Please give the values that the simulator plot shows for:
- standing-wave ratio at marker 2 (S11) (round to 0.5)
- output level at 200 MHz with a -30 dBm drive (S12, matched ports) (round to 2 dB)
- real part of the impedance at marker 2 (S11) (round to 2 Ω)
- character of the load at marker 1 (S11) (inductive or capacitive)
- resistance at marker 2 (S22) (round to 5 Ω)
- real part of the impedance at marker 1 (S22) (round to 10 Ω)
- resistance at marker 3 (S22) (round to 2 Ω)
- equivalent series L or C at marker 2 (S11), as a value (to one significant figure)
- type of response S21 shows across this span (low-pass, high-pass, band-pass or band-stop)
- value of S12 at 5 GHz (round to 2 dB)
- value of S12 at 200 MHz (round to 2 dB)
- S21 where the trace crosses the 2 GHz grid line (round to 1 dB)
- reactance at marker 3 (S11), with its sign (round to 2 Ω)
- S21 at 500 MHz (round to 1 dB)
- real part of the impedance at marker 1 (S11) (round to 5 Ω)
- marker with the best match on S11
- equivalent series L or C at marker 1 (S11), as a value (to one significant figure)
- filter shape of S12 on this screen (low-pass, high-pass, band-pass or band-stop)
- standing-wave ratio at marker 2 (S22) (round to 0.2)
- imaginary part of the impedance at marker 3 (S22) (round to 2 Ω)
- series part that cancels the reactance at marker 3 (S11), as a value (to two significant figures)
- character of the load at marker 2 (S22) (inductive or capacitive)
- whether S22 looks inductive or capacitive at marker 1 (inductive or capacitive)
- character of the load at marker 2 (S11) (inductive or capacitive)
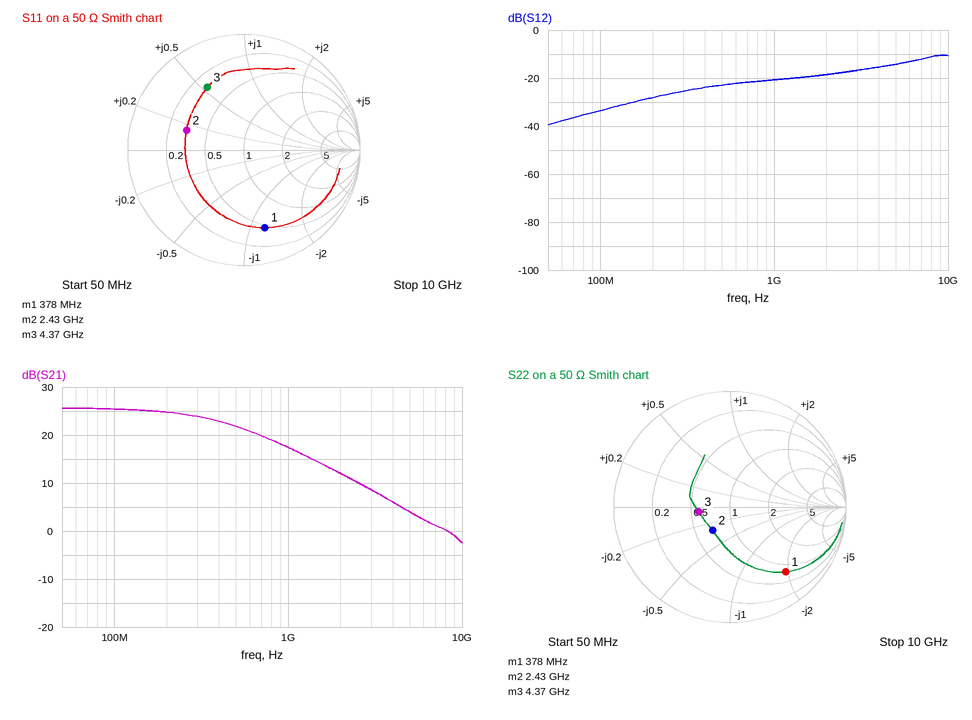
3.0
-58 dBm
16 Ω
capacitive
35 Ω
40 Ω
28 Ω
500 pH
low-pass
-14 dB
-28 dB
12 dB
+26 Ω
22 dB
25 Ω
marker 2
7 pF
high-pass
1.6
-2 Ω
1.4 pF
capacitive
capacitive
inductive
